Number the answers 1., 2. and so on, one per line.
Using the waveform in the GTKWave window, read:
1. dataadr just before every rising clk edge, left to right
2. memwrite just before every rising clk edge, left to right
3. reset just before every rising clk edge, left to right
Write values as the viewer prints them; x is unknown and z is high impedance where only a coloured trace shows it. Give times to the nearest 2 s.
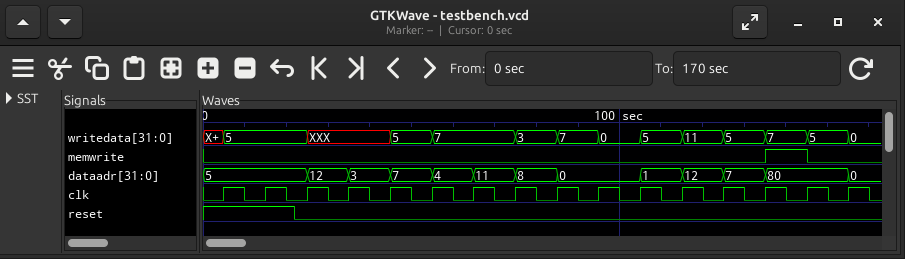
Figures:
1. 5, 5, 5, 12, 3, 7, 4, 11, 8, 0, 0, 1, 12, 7, 80, 80
2. 0 0 0 0 0 0 0 0 0 0 0 0 0 0 1 0
3. 1 1 0 0 0 0 0 0 0 0 0 0 0 0 0 0
